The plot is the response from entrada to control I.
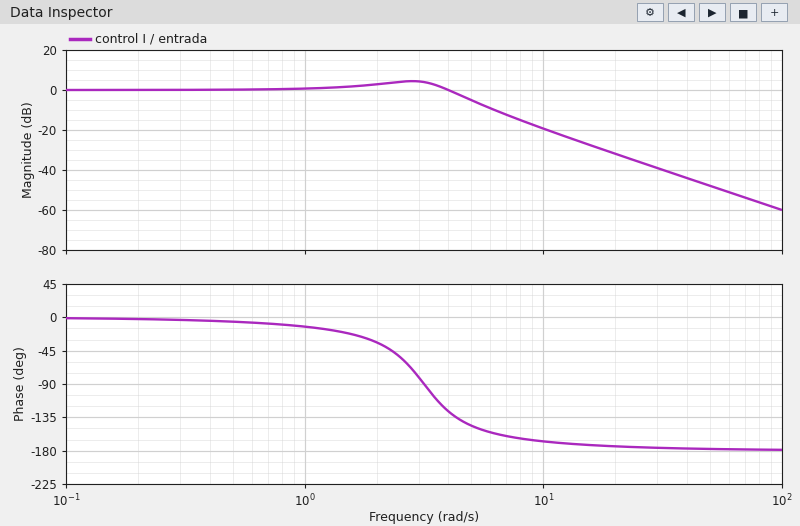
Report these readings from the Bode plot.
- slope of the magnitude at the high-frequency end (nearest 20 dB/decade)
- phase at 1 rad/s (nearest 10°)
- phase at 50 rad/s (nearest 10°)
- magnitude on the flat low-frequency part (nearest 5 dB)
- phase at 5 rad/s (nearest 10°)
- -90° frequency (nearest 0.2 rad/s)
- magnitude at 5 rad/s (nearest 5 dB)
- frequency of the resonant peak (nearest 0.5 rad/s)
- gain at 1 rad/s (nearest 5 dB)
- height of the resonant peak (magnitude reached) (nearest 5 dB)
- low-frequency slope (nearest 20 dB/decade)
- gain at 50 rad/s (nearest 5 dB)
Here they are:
-40 dB/decade
-10°
-180°
0 dB
-150°
3.2 rad/s
-5 dB
3.0 rad/s
0 dB
5 dB
0 dB/decade
-50 dB
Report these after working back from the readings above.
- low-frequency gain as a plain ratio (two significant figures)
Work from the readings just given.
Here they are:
1.0
